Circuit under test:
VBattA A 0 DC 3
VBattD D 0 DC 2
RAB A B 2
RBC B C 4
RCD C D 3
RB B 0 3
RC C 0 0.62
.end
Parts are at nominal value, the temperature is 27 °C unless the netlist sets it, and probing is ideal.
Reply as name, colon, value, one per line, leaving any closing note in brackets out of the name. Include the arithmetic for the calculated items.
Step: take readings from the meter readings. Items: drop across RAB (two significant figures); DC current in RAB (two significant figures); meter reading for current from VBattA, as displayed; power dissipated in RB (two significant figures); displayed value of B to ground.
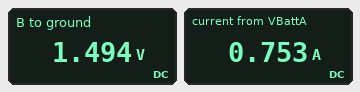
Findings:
drop across RAB: 3 V - 1.494 V = 1.5 V
DC current in RAB: (3 V - 1.494 V) / 2 Ω = 750 mA
meter reading for current from VBattA, as displayed: 0.753 A
power dissipated in RB: (1.494 V)^2 / 3 Ω = 740 mW
displayed value of B to ground: 1.494 V
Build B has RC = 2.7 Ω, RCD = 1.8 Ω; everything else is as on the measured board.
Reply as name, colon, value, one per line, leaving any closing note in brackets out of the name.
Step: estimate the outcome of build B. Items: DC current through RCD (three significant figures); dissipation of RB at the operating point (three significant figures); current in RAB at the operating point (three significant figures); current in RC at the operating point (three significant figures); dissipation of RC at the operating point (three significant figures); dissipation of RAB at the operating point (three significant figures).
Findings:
DC current through RCD: 387 mA
dissipation of RB at the operating point: 947 mW
current in RAB at the operating point: 657 mA
current in RC at the operating point: 483 mA
dissipation of RC at the operating point: 629 mW
dissipation of RAB at the operating point: 864 mW
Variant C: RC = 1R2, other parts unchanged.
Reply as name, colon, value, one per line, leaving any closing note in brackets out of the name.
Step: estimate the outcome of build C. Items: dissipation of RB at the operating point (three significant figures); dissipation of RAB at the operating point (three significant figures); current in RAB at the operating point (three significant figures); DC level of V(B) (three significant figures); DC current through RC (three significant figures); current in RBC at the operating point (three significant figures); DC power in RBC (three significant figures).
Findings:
dissipation of RB at the operating point: 808 mW
dissipation of RAB at the operating point: 1.04 W
current in RAB at the operating point: 722 mA
DC level of V(B): 1.56 V
DC current through RC: 621 mA
current in RBC at the operating point: 203 mA
DC power in RBC: 165 mW
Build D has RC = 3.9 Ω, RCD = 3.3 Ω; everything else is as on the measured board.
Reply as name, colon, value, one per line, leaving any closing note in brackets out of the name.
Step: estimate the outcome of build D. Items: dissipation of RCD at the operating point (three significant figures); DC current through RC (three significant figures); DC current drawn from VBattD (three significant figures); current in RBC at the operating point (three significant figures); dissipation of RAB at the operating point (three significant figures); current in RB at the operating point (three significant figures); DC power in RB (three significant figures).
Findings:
dissipation of RCD at the operating point: 163 mW
DC current through RC: 325 mA
DC current drawn from VBattD: 222 mA
current in RBC at the operating point: 103 mA
dissipation of RAB at the operating point: 875 mW
current in RB at the operating point: 559 mA
DC power in RB: 937 mW
